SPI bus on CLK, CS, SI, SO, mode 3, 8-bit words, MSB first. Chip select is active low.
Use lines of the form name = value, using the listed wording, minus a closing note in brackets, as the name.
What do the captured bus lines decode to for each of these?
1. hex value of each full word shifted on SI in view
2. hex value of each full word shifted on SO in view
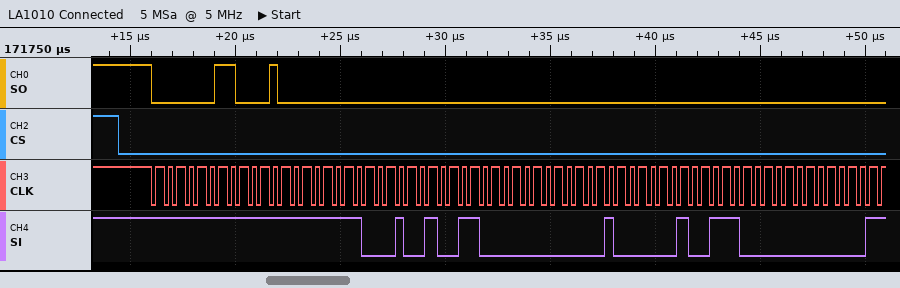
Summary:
hex value of each full word shifted on SI in view = FF, FF, F1, 26, 00, 10, 27, 00
hex value of each full word shifted on SO in view = 03, 10, 00, 00, 00, 00, 00, 00
